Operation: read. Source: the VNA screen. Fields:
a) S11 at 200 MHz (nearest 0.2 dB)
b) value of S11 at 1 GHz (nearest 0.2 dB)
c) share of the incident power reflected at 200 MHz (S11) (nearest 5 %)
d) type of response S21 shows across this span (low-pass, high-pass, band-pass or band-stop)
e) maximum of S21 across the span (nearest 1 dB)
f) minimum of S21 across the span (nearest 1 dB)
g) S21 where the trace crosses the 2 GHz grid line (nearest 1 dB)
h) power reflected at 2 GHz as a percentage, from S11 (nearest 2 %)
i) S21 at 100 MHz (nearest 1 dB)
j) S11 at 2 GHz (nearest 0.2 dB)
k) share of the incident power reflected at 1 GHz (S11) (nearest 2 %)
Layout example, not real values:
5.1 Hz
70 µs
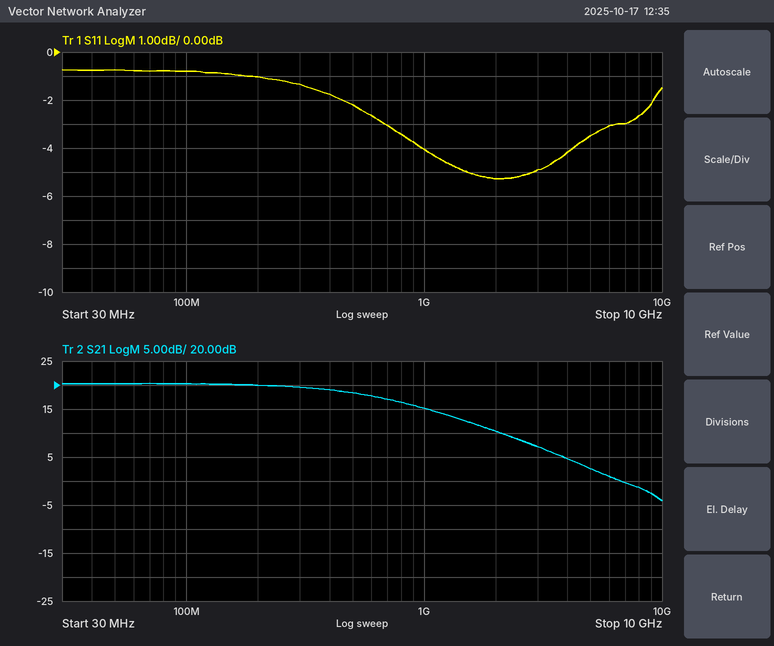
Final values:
-1.0 dB
-4.0 dB
80 %
low-pass
20 dB
-4 dB
10 dB
30 %
20 dB
-5.2 dB
40 %
